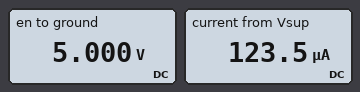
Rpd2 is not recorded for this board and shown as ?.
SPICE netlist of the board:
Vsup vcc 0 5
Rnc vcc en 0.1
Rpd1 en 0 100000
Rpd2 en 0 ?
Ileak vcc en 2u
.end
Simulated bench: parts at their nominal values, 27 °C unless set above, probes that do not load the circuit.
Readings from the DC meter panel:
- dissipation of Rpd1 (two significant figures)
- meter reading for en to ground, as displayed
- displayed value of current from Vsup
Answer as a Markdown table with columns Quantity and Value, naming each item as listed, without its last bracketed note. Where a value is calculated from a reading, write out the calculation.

| Quantity | Value |
|---|---|
| dissipation of Rpd1 | (5 V)^2 / 100 kΩ = 250 µW |
| meter reading for en to ground, as displayed | 5.000 V |
| displayed value of current from Vsup | 123.5 µA |
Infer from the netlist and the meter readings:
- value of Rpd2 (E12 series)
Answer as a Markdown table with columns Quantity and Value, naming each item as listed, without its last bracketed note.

| Quantity | Value |
|---|---|
| value of Rpd2 | 68 kΩ |
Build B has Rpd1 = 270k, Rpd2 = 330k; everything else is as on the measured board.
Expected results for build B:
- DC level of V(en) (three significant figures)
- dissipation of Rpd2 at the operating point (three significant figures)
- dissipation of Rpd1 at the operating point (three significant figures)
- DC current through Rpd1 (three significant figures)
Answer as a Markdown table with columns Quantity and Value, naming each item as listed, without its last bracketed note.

| Quantity | Value |
|---|---|
| DC level of V(en) | 5.00 V |
| dissipation of Rpd2 at the operating point | 75.8 µW |
| dissipation of Rpd1 at the operating point | 92.6 µW |
| DC current through Rpd1 | 18.5 µA |
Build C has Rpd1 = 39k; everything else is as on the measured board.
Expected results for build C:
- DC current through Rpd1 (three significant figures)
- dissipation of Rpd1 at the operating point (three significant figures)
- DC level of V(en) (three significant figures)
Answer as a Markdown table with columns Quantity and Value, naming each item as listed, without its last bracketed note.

| Quantity | Value |
|---|---|
| DC current through Rpd1 | 128 µA |
| dissipation of Rpd1 at the operating point | 641 µW |
| DC level of V(en) | 5.00 V |
